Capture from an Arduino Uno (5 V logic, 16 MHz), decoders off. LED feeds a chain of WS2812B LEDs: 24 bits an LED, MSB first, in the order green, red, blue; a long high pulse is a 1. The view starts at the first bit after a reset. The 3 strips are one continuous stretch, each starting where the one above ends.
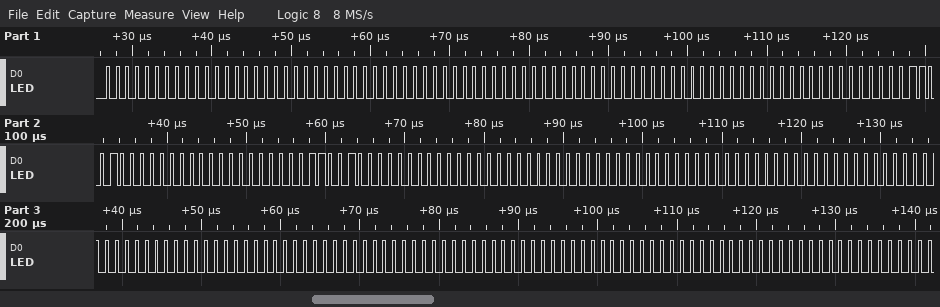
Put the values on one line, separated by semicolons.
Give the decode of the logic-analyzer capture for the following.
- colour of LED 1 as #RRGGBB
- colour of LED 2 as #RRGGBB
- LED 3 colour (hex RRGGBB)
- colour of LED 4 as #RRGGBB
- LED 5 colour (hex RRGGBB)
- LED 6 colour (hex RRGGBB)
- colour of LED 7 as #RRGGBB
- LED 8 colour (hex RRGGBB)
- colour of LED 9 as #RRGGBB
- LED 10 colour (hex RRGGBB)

#000000; #000000; #000000; #640000; #640000; #000000; #000000; #000000; #000000; #000000
